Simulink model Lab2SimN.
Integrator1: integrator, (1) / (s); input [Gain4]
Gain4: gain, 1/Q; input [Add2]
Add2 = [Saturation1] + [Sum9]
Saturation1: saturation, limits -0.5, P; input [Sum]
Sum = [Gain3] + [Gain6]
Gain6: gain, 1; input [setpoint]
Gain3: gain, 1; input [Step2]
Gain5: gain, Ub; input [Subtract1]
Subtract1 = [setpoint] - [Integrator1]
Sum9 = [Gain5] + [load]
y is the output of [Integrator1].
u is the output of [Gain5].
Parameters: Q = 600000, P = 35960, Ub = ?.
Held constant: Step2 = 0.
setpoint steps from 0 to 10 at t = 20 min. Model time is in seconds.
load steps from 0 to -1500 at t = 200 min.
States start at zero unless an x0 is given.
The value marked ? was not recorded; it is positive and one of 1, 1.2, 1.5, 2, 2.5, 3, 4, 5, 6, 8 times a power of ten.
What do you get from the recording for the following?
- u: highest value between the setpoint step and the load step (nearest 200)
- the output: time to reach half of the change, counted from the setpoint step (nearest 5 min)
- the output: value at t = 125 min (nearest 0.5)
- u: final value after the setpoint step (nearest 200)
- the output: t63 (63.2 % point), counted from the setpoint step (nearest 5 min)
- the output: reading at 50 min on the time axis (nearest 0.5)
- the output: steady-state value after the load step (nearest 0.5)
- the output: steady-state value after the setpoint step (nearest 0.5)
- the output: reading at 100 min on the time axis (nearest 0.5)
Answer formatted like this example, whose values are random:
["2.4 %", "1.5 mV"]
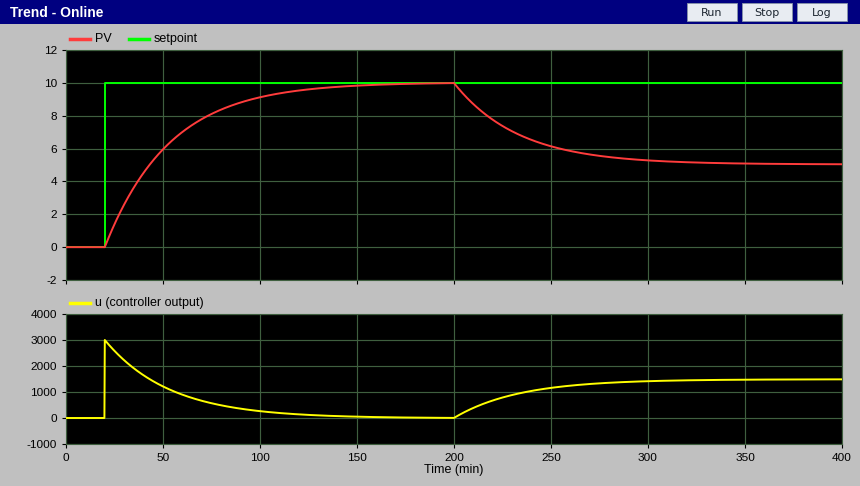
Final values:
["3000", "25 min", "9.5", "0", "35 min", "6.0", "5.0", "10.0", "9.0"]
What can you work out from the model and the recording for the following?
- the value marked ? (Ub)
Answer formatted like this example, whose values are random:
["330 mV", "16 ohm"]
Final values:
["300"]
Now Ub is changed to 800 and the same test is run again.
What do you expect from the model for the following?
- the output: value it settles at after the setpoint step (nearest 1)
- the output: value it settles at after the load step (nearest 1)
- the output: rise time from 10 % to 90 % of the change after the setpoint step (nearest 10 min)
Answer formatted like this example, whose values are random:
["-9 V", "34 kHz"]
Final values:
["10", "8", "30 min"]
